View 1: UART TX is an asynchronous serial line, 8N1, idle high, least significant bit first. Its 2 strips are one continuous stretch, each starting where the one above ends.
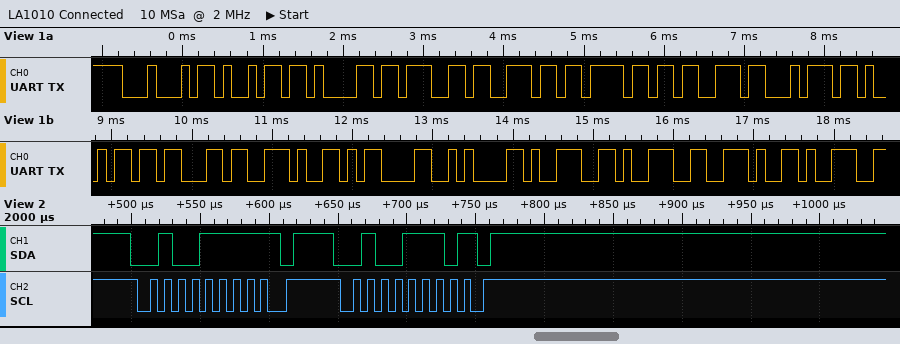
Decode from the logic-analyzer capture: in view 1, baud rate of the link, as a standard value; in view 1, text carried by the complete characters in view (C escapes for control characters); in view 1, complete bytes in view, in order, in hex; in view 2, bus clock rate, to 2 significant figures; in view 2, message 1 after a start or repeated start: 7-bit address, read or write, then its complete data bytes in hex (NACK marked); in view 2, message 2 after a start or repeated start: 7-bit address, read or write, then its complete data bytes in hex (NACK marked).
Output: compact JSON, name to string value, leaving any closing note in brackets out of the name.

{"in view 1, baud rate of the link, as a standard value": "9600 baud", "in view 1, text carried by the complete characters in view": "\"Diagnostic.\\r\\n99.9\"", "in view 1, complete bytes in view, in order, in hex": "0x44 0x69 0x61 0x67 0x6E 0x6F 0x73 0x74 0x69 0x63 0x2E 0x0D 0x0A 0x39 0x39 0x2E 0x39", "in view 2, bus clock rate, to 2 significant figures": "100 kHz", "in view 2, message 1 after a start or repeated start: 7-bit address, read or write, then its complete data bytes in hex": "0x27 read NACK", "in view 2, message 2 after a start or repeated start: 7-bit address, read or write, then its complete data bytes in hex": "0x27 write NACK"}
